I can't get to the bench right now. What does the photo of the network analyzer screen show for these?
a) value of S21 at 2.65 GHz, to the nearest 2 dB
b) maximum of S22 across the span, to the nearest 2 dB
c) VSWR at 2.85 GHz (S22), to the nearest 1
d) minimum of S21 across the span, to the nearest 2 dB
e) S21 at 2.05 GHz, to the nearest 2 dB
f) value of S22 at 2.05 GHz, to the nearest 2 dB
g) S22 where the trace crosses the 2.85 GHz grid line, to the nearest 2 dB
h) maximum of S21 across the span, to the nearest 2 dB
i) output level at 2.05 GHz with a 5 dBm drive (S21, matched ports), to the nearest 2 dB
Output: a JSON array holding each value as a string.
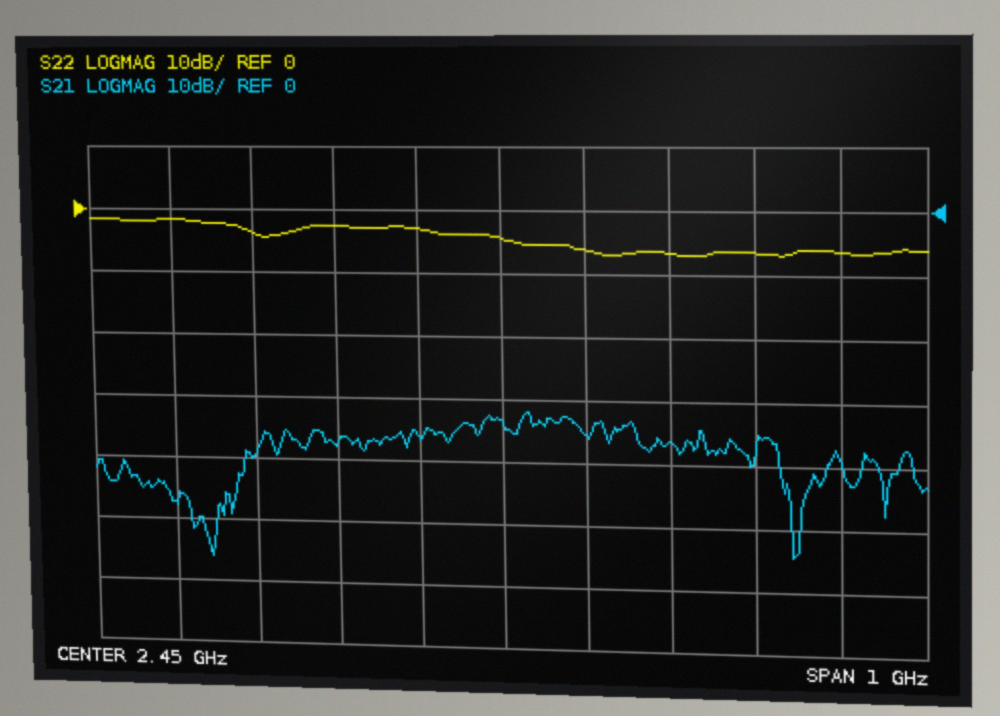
["-36 dB", "-2 dB", "3", "-56 dB", "-48 dB", "-2 dB", "-6 dB", "-32 dB", "-42 dBm"]
